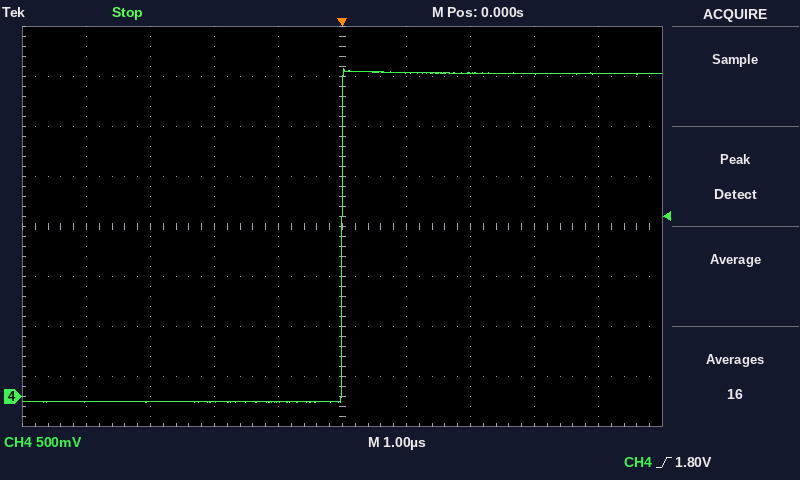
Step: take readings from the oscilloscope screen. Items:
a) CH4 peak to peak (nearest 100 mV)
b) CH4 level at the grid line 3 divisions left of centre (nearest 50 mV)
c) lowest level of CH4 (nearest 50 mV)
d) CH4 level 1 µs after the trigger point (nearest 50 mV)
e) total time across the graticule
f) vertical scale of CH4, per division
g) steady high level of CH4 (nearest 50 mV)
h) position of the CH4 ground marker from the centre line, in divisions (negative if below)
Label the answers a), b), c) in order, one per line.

a) 3.30 V
b) -50 mV
c) -50 mV
d) 3.25 V
e) 10 µs
f) 500 mV
g) 3.25 V
h) -3.4 div
